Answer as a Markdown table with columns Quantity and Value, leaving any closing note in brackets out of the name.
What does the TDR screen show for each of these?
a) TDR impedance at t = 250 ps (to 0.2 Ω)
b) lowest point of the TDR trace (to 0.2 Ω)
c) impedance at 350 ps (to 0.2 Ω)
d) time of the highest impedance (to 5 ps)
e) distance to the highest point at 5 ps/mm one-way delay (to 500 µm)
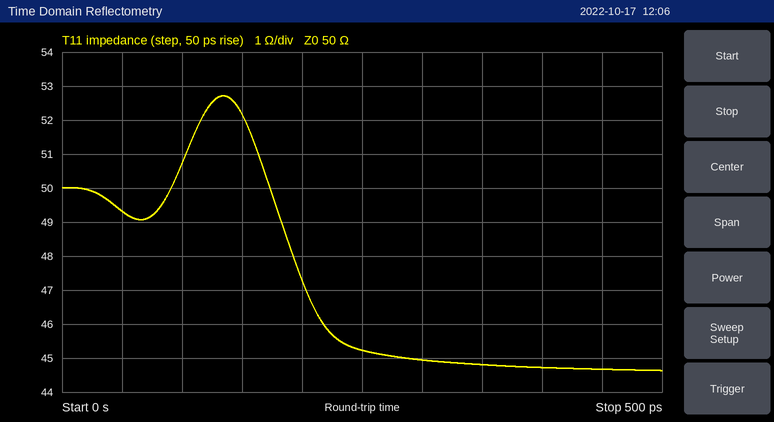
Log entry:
| Quantity | Value |
|---|---|
| TDR impedance at t = 250 ps | 45.2 Ω |
| lowest point of the TDR trace | 44.6 Ω |
| impedance at 350 ps | 44.8 Ω |
| time of the highest impedance | 135 ps |
| distance to the highest point at 5 ps/mm one-way delay | 13.5 mm |
